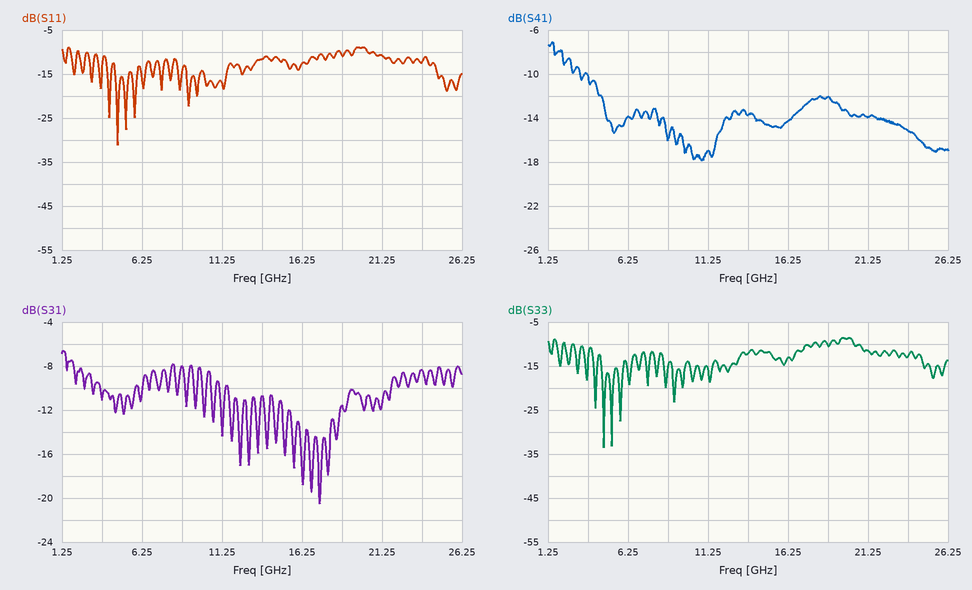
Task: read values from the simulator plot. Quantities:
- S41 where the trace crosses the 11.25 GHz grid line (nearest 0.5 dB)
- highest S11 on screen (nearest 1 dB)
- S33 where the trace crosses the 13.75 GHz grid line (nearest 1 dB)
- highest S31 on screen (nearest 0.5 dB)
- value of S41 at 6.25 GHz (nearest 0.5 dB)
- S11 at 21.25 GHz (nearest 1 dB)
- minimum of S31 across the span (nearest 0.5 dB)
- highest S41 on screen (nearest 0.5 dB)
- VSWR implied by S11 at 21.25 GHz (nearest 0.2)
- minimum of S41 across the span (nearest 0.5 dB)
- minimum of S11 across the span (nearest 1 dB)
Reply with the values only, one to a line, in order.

-17.0 dB
-9 dB
-12 dB
-6.5 dB
-14.0 dB
-11 dB
-20.5 dB
-7.0 dB
1.8
-18.0 dB
-31 dB
